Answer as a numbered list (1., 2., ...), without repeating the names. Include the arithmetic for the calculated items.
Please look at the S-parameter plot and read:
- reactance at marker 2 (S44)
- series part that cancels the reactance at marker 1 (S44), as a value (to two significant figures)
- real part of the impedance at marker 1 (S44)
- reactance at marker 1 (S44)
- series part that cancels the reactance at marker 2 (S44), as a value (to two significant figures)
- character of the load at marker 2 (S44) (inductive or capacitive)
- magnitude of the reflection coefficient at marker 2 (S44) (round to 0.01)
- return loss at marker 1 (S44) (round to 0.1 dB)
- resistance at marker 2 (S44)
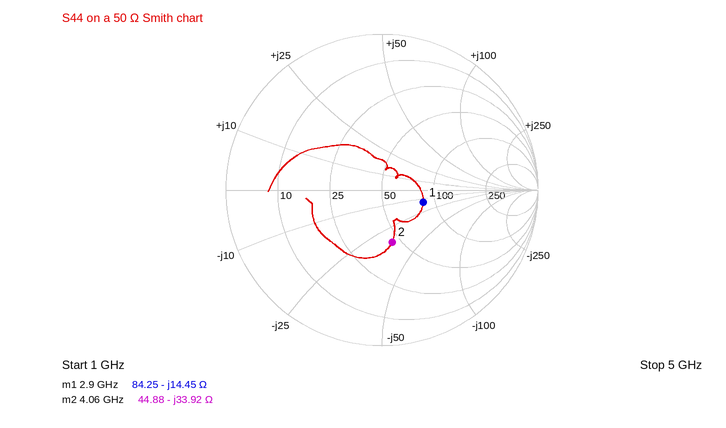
1. -33.92 Ω
2. L = 14.45 Ω/(2π × 2.9 GHz) ≈ 793 pH, so 790 pH to two significant figures
3. 84.25 Ω
4. -14.45 Ω
5. L = 33.92 Ω/(2π × 4.06 GHz) ≈ 1.3 nH
6. capacitive
7. 0.34
8. 11.2 dB
9. 44.88 Ω
